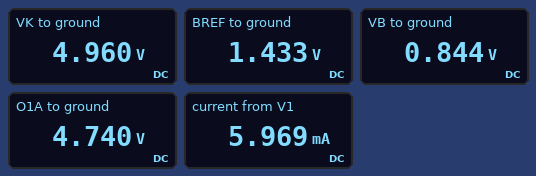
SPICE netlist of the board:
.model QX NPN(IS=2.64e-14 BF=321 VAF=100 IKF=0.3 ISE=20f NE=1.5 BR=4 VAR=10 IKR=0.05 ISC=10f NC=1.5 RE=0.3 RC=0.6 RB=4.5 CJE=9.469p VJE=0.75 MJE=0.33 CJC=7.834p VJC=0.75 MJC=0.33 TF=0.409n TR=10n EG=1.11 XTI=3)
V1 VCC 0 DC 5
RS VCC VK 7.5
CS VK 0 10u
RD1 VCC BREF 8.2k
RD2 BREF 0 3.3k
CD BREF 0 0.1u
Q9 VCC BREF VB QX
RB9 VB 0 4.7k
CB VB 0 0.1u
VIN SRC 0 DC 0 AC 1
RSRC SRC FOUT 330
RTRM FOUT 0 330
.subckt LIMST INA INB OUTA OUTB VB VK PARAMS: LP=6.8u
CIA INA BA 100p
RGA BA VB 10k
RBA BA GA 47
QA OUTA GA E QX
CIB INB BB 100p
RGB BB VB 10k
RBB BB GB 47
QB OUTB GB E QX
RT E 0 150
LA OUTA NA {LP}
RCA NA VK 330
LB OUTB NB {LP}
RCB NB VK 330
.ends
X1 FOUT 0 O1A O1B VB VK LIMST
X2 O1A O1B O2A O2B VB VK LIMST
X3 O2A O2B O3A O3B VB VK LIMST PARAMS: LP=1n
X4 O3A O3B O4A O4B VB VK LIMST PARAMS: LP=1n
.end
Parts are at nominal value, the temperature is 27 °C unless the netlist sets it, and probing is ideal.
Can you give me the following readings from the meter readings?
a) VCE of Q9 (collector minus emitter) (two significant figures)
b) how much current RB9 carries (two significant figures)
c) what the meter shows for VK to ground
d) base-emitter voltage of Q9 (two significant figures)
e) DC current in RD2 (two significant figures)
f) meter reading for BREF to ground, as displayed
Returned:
4.2 V
180 µA
4.960 V
590 mV
430 µA
1.433 V
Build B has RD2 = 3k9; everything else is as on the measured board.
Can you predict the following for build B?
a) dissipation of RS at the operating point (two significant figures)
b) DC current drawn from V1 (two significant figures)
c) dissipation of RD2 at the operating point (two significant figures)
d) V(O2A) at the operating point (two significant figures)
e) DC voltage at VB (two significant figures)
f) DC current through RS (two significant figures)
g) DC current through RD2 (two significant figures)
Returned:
620 µW
9.7 mA
660 µW
4.6 V
1.0 V
9.1 mA
410 µA
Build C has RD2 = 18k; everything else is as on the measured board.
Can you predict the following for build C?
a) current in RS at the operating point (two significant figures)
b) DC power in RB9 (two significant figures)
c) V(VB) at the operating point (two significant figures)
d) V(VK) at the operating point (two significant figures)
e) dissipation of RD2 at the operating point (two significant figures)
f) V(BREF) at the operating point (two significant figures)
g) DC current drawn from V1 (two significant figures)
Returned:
50 mA
1.7 mW
2.8 V
4.6 V
650 µW
3.4 V
51 mA
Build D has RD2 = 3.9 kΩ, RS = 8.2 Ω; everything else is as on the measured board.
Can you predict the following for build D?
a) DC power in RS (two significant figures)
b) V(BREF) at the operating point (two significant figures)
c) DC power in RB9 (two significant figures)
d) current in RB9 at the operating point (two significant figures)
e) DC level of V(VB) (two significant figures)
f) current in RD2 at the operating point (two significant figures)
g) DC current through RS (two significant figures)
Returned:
670 µW
1.6 V
220 µW
220 µA
1.0 V
410 µA
9.1 mA
